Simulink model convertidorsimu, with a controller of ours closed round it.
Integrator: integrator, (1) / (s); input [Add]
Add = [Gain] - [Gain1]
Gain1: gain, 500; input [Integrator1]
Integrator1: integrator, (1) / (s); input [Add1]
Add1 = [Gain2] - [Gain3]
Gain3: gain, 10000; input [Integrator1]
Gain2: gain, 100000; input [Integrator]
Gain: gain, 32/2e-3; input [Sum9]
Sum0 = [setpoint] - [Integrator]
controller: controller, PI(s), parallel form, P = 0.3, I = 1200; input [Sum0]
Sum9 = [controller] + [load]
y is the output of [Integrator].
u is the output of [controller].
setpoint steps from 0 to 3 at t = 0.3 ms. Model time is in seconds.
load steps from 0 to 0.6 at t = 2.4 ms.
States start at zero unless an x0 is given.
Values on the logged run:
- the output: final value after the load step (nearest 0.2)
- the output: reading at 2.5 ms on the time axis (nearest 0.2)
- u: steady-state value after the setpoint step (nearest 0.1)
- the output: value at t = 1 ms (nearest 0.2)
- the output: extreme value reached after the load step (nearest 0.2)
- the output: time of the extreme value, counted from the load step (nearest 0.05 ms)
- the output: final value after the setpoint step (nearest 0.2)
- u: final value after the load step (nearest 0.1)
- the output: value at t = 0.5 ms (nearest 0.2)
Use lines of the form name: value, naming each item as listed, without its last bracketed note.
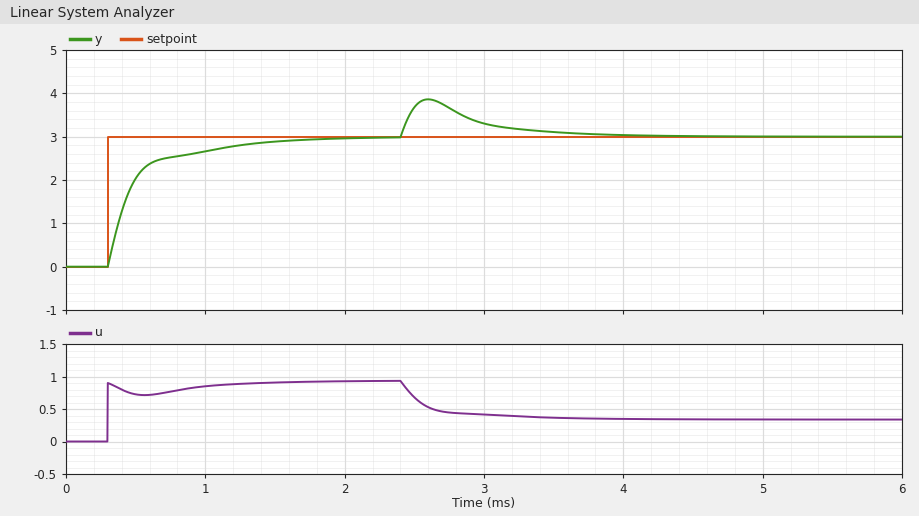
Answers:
the output: final value after the load step: 3.0
the output: reading at 2.5 ms on the time axis: 3.6
u: steady-state value after the setpoint step: 0.9
the output: value at t = 1 ms: 2.6
the output: extreme value reached after the load step: 3.8
the output: time of the extreme value, counted from the load step: 0.20 ms
the output: final value after the setpoint step: 3.0
u: final value after the load step: 0.3
the output: value at t = 0.5 ms: 2.0
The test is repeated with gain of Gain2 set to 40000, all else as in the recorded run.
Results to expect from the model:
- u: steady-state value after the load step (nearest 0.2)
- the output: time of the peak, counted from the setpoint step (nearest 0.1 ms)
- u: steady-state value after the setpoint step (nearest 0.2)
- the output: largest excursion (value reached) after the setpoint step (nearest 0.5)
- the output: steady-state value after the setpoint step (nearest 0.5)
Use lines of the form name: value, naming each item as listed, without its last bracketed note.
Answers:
u: steady-state value after the load step: -0.2
the output: time of the peak, counted from the setpoint step: 0.5 ms
u: steady-state value after the setpoint step: 0.4
the output: largest excursion (value reached) after the setpoint step: 3.0
the output: steady-state value after the setpoint step: 3.0
